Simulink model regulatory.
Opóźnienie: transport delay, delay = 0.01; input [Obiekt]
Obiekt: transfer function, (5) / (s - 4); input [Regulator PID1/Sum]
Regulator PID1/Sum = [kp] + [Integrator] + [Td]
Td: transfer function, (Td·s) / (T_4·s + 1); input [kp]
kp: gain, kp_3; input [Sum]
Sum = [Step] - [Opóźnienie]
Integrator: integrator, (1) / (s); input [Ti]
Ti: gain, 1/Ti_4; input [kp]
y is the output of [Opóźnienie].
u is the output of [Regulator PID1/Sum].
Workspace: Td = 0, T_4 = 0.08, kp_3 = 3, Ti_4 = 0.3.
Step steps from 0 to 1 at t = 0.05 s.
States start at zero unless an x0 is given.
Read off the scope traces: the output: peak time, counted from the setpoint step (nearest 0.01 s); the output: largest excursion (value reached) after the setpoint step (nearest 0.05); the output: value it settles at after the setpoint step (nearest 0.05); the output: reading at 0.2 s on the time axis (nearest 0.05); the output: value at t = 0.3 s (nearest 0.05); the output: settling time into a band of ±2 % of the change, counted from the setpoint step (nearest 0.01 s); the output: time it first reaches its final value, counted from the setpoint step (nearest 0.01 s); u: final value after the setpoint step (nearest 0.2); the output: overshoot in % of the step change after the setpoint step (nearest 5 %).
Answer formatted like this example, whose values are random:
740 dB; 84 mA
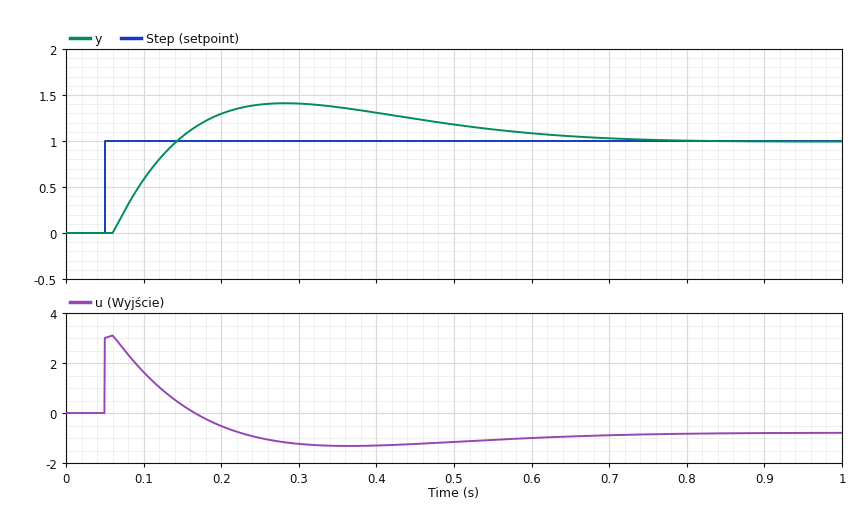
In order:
0.23 s; 1.40; 1.00; 1.30; 1.40; 0.68 s; 0.09 s; -0.8; 40 %
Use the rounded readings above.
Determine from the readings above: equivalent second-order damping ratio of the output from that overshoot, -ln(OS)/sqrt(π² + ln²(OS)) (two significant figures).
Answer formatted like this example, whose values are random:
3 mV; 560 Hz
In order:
0.28
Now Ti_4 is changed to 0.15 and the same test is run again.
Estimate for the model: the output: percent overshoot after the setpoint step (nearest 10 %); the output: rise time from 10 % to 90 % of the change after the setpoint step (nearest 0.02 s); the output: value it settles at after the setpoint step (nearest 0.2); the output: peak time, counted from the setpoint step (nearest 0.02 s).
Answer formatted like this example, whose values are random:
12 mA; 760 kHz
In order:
50 %; 0.06 s; 1.0; 0.20 s
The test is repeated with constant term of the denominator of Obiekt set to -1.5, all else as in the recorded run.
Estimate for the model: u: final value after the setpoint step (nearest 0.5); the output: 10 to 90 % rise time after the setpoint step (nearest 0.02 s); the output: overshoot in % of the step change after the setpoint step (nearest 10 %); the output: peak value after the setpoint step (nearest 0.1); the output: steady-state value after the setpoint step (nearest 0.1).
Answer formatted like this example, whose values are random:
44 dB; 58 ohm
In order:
-0.5; 0.08 s; 20 %; 1.2; 1.0
